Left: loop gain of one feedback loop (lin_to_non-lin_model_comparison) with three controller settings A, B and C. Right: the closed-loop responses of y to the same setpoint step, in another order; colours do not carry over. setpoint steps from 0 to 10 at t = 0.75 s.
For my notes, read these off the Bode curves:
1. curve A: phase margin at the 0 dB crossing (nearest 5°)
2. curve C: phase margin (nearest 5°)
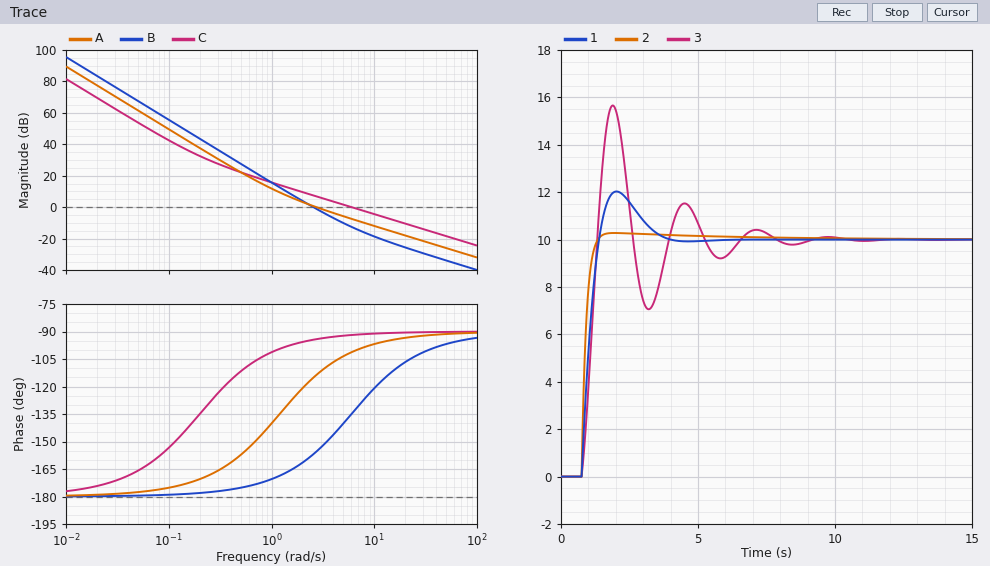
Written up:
65°
90°
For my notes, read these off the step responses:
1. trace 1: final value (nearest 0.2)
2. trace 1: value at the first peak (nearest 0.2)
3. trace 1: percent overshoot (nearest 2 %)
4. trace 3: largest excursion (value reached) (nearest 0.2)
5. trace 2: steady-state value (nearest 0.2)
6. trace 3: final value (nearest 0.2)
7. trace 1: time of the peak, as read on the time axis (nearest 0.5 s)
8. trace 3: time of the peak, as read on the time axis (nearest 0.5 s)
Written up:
10.0
12.0
20 %
15.6
10.0
10.0
2.0 s
2.0 s
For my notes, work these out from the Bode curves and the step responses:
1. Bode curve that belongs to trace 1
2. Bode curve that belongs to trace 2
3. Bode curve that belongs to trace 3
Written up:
A
C
B
